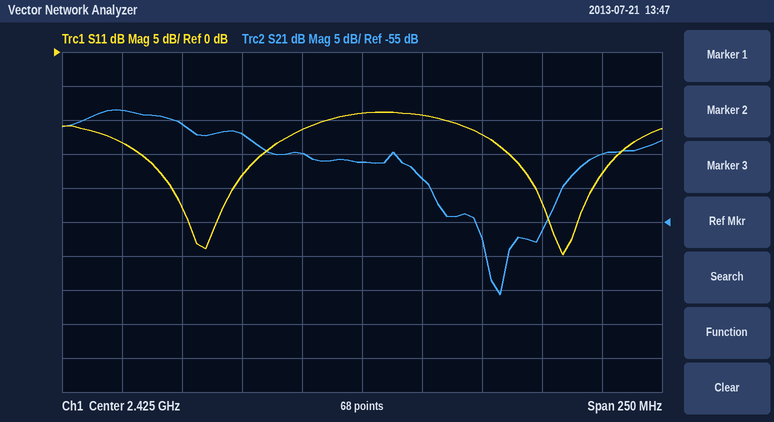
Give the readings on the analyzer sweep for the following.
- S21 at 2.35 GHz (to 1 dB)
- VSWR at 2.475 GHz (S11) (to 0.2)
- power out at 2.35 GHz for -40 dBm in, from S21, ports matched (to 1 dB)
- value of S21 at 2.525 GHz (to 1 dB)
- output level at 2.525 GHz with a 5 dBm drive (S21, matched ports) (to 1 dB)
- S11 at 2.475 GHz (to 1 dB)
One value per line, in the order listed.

-41 dB
1.6
-81 dBm
-45 dB
-40 dBm
-12 dB
